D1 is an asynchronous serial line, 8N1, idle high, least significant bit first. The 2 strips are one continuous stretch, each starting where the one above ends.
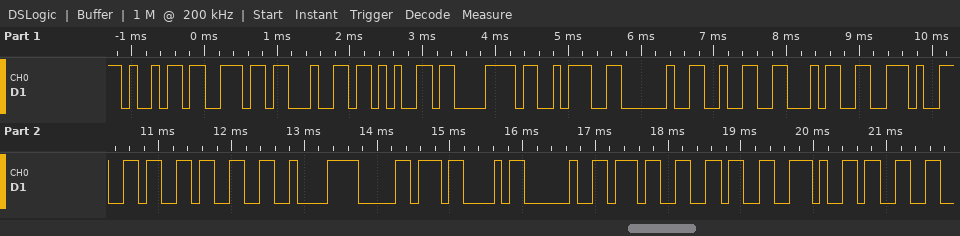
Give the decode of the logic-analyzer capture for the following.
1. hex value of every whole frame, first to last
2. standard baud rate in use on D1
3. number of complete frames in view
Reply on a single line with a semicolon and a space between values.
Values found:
0x69 0x6E 0x64 0x65 0x78 0x3A 0x20 0x32 0x34 0x2E 0x36 0x33 0xC2 0xB0 0x43 0x20 0x37 0x36 0x2E 0x33; 9600 baud; 20
